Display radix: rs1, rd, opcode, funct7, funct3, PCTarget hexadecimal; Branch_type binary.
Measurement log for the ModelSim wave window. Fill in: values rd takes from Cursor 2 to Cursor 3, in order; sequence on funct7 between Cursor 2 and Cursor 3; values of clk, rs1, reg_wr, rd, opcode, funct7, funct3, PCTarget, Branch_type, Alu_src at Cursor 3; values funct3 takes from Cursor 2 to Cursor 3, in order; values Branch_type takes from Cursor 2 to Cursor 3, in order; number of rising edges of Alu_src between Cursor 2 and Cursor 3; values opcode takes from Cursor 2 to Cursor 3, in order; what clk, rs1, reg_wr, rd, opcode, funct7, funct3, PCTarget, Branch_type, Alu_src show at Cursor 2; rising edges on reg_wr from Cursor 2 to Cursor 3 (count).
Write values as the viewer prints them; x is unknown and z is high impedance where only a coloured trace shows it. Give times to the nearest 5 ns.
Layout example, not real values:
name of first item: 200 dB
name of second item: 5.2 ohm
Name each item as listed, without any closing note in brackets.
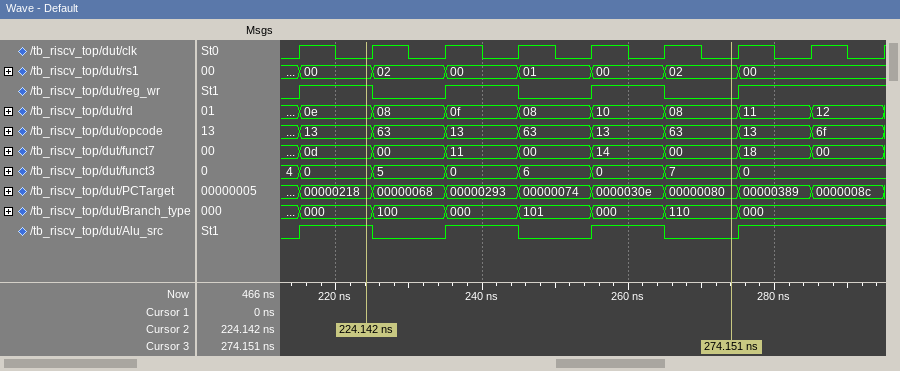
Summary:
values rd takes from Cursor 2 to Cursor 3, in order: 0e, 08, 0f, 08, 10, 08
sequence on funct7 between Cursor 2 and Cursor 3: 0d, 00, 11, 00, 14, 00
values of clk, rs1, reg_wr, rd, opcode, funct7, funct3, PCTarget, Branch_type, Alu_src at Cursor 3: clk=0, rs1=02, reg_wr=0, rd=08, opcode=63, funct7=00, funct3=7, PCTarget=00000080, Branch_type=110, Alu_src=0
values funct3 takes from Cursor 2 to Cursor 3, in order: 0, 5, 0, 6, 0, 7
values Branch_type takes from Cursor 2 to Cursor 3, in order: 000, 100, 000, 101, 000, 110
number of rising edges of Alu_src between Cursor 2 and Cursor 3: 2
values opcode takes from Cursor 2 to Cursor 3, in order: 13, 63, 13, 63, 13, 63
what clk, rs1, reg_wr, rd, opcode, funct7, funct3, PCTarget, Branch_type, Alu_src show at Cursor 2: clk=0, rs1=00, reg_wr=1, rd=0e, opcode=13, funct7=0d, funct3=0, PCTarget=00000218, Branch_type=000, Alu_src=1
rising edges on reg_wr from Cursor 2 to Cursor 3: 2
